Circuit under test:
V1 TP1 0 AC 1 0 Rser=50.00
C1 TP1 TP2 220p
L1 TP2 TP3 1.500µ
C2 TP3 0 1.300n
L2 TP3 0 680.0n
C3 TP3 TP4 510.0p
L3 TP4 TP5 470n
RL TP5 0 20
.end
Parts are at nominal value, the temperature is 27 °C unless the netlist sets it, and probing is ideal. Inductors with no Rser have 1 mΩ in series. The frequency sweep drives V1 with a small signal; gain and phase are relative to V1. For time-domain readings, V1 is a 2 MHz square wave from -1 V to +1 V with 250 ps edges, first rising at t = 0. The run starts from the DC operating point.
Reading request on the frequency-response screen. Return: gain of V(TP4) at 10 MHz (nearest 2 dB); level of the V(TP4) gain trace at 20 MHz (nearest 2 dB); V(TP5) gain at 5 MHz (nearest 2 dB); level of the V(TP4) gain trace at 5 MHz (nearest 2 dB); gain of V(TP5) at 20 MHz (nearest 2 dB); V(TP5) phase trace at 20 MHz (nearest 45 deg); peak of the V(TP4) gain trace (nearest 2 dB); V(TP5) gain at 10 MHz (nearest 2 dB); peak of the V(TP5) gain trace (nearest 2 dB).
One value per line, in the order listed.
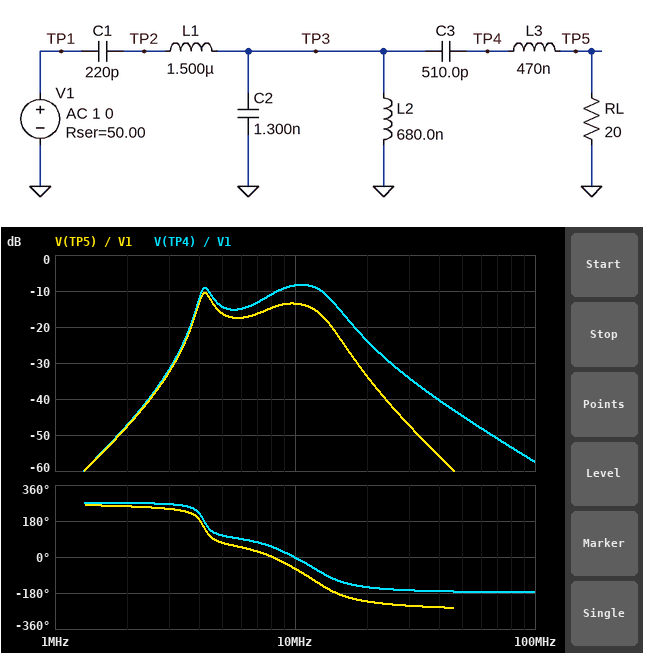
-8 dB
-24 dB
-16 dB
-14 dB
-34 dB
-225 deg
-8 dB
-14 dB
-10 dB
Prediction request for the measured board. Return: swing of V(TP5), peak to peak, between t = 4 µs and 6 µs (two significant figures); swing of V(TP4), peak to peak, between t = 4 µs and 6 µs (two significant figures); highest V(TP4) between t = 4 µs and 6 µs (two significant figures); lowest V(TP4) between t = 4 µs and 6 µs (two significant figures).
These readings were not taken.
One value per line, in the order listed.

250 mV
430 mV
220 mV
-220 mV
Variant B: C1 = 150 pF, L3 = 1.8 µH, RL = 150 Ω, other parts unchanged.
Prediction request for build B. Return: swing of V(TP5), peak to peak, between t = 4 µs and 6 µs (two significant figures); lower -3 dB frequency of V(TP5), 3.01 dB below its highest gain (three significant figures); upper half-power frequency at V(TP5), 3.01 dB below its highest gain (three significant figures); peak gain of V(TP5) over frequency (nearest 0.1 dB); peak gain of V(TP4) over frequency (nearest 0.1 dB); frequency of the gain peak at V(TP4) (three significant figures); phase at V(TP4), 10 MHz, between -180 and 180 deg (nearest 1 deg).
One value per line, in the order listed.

480 mV
4.64 MHz
5.64 MHz
-3.1 dB
-2.5 dB
5.05 MHz
-46 deg
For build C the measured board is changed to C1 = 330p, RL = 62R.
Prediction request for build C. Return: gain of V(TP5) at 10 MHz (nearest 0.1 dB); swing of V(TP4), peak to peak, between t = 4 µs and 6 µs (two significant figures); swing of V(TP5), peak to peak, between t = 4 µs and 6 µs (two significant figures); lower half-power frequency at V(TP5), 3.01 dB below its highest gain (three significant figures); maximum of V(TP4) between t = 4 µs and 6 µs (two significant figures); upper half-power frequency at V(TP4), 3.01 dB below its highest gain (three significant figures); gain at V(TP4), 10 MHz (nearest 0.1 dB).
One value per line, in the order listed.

-11.6 dB
500 mV
470 mV
3.89 MHz
250 mV
8.34 MHz
-10.7 dB
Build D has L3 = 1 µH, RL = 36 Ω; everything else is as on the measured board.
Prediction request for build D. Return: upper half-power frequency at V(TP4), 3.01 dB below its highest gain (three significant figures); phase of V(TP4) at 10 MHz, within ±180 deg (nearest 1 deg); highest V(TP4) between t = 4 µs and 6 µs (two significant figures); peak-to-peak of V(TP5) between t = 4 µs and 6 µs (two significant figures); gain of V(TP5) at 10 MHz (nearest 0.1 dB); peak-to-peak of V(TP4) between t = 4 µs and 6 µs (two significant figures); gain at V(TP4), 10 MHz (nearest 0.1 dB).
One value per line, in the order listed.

11.1 MHz
-54 deg
330 mV
380 mV
-11.1 dB
650 mV
-5.0 dB
